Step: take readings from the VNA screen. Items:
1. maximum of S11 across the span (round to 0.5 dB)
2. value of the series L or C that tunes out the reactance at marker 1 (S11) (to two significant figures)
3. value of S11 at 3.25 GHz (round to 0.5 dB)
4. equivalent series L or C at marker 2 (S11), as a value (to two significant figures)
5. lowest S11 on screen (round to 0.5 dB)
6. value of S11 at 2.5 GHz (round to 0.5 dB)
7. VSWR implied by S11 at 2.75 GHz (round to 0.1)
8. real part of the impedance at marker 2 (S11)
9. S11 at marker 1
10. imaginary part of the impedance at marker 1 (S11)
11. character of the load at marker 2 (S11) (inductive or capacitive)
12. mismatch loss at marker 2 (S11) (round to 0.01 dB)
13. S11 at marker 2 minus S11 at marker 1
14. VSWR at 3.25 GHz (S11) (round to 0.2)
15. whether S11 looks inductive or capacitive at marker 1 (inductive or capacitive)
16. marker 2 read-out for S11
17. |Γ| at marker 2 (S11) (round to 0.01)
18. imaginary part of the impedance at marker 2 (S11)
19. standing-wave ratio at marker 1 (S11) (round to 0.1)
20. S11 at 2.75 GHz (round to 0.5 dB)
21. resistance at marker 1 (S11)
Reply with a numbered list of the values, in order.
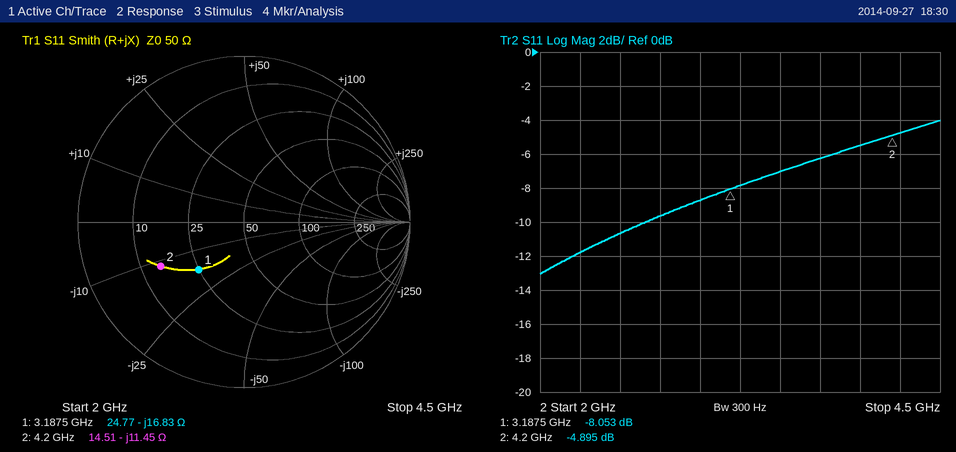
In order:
1. -4.0 dB
2. 840 pH
3. -8.0 dB
4. 3.3 pF
5. -13.0 dB
6. -10.5 dB
7. 2.0
8. 14.51 Ω
9. -8.053 dB
10. -16.83 Ω
11. capacitive
12. 1.70 dB
13. 3.158 dB
14. 2.4
15. capacitive
16. -4.895 dB
17. 0.57
18. -11.45 Ω
19. 2.3
20. -9.5 dB
21. 24.77 Ω
